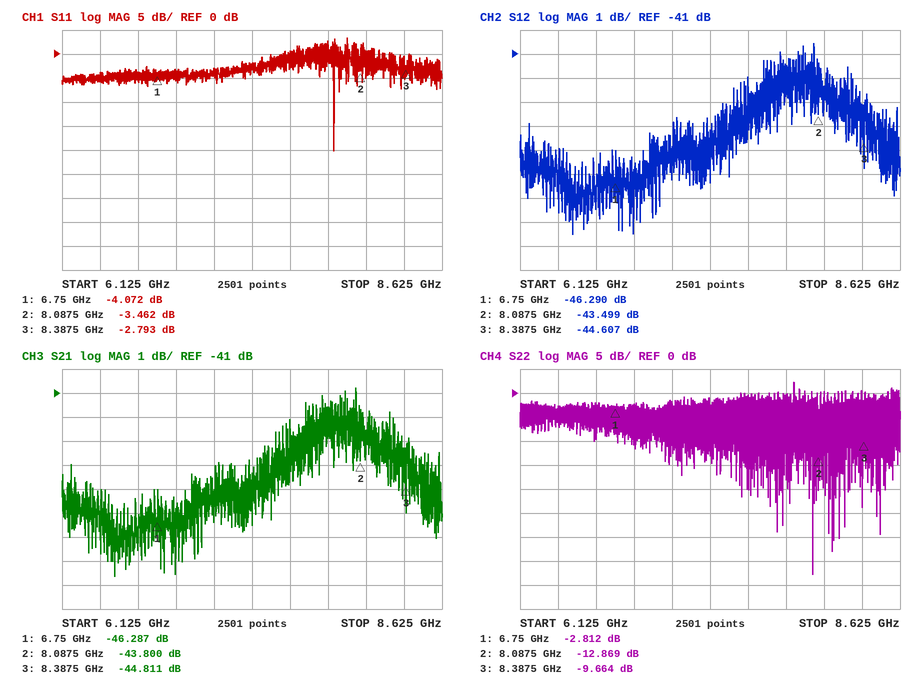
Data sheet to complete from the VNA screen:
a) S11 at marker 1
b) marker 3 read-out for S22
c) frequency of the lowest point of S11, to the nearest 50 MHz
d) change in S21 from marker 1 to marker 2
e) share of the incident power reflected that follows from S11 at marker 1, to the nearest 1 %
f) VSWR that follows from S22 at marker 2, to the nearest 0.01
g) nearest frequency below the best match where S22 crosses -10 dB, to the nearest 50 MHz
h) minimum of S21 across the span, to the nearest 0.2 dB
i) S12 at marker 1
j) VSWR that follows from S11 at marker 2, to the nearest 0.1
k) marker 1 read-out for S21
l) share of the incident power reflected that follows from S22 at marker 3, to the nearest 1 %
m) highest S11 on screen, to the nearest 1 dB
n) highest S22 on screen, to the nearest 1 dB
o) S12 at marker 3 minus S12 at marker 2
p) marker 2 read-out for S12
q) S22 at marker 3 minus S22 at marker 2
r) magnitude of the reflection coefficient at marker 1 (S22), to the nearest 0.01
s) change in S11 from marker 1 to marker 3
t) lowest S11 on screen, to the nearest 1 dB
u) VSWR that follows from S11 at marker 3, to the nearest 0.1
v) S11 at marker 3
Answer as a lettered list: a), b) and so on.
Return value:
a) -4.072 dB
b) -9.664 dB
c) 7.90 GHz
d) 2.487 dB
e) 39 %
f) 1.59
g) 8.05 GHz
h) -48.6 dB
i) -46.290 dB
j) 5.1
k) -46.287 dB
l) 11 %
m) 3 dB
n) 2 dB
o) -1.108 dB
p) -43.499 dB
q) 3.205 dB
r) 0.72
s) 1.279 dB
t) -20 dB
u) 6.3
v) -2.793 dB
